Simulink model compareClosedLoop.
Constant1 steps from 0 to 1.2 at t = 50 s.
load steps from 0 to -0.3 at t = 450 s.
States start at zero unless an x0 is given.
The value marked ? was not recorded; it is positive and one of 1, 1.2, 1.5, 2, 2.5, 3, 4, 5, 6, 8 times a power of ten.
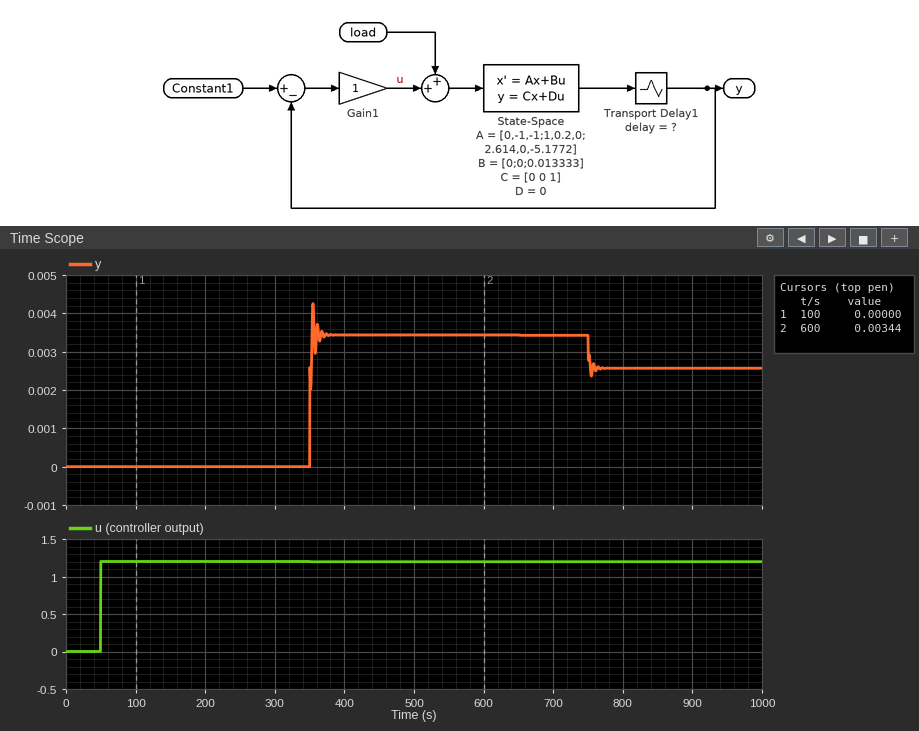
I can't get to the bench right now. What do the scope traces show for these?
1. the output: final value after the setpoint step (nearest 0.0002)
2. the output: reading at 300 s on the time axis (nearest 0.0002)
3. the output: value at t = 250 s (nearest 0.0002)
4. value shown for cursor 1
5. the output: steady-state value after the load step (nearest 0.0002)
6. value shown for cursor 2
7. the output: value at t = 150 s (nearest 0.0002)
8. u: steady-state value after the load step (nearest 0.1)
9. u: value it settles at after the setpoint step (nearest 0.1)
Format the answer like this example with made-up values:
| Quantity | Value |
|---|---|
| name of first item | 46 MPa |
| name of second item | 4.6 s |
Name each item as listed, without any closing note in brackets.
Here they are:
| Quantity | Value |
|---|---|
| the output: final value after the setpoint step | 0.0034 |
| the output: reading at 300 s on the time axis | 0.0000 |
| the output: value at t = 250 s | 0.0000 |
| value shown for cursor 1 | 0.00000 |
| the output: steady-state value after the load step | 0.0026 |
| value shown for cursor 2 | 0.00344 |
| the output: value at t = 150 s | 0.0000 |
| u: steady-state value after the load step | 1.2 |
| u: value it settles at after the setpoint step | 1.2 |
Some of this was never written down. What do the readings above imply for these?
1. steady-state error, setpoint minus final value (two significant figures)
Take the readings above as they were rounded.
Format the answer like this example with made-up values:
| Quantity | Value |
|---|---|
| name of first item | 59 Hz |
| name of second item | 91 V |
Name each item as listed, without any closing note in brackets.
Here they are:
| Quantity | Value |
|---|---|
| steady-state error, setpoint minus final value | 1.2 |
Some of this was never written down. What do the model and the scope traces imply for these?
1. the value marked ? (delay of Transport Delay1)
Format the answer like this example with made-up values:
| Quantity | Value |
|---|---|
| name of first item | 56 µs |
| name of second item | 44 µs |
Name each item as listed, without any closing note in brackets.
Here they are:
| Quantity | Value |
|---|---|
| the value marked ? | 300 |
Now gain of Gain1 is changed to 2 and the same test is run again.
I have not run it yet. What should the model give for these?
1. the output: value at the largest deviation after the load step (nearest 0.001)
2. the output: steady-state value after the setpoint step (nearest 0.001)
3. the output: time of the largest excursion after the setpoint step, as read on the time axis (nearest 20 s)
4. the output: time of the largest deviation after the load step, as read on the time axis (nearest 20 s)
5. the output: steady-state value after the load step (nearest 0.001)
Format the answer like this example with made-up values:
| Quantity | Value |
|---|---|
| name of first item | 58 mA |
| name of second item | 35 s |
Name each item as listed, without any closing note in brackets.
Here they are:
| Quantity | Value |
|---|---|
| the output: value at the largest deviation after the load step | 0.006 |
| the output: steady-state value after the setpoint step | 0.007 |
| the output: time of the largest excursion after the setpoint step, as read on the time axis | 360 s |
| the output: time of the largest deviation after the load step, as read on the time axis | 760 s |
| the output: steady-state value after the load step | 0.006 |
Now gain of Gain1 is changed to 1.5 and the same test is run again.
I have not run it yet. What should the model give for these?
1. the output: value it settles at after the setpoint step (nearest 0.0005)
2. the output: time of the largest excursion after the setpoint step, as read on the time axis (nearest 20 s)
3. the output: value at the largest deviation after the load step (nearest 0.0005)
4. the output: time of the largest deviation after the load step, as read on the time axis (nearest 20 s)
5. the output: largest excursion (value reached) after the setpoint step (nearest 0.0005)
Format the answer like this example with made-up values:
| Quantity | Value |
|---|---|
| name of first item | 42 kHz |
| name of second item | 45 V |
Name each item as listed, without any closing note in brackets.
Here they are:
| Quantity | Value |
|---|---|
| the output: value it settles at after the setpoint step | 0.0050 |
| the output: time of the largest excursion after the setpoint step, as read on the time axis | 360 s |
| the output: value at the largest deviation after the load step | 0.0040 |
| the output: time of the largest deviation after the load step, as read on the time axis | 760 s |
| the output: largest excursion (value reached) after the setpoint step | 0.0065 |
